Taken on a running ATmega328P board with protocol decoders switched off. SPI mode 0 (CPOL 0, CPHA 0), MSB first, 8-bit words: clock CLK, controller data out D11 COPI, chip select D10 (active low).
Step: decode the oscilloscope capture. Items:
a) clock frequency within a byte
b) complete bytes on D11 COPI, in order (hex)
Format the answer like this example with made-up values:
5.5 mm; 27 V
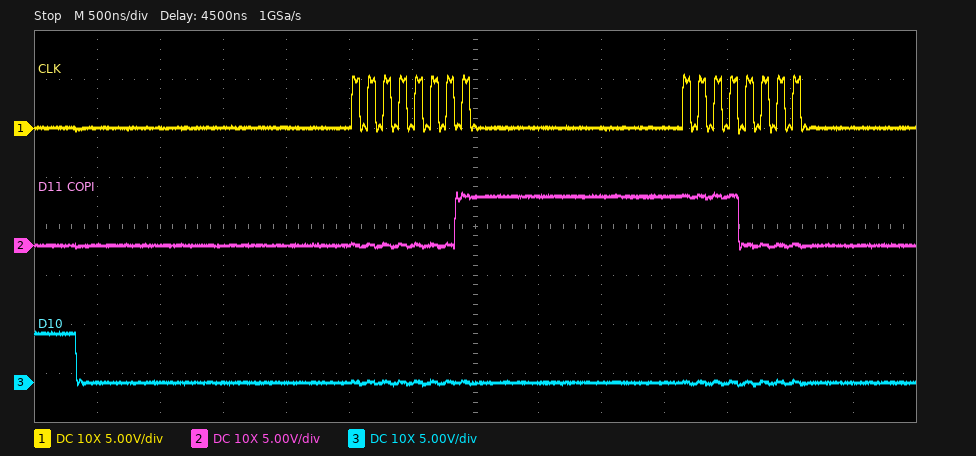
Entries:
8 MHz; 01 F0
